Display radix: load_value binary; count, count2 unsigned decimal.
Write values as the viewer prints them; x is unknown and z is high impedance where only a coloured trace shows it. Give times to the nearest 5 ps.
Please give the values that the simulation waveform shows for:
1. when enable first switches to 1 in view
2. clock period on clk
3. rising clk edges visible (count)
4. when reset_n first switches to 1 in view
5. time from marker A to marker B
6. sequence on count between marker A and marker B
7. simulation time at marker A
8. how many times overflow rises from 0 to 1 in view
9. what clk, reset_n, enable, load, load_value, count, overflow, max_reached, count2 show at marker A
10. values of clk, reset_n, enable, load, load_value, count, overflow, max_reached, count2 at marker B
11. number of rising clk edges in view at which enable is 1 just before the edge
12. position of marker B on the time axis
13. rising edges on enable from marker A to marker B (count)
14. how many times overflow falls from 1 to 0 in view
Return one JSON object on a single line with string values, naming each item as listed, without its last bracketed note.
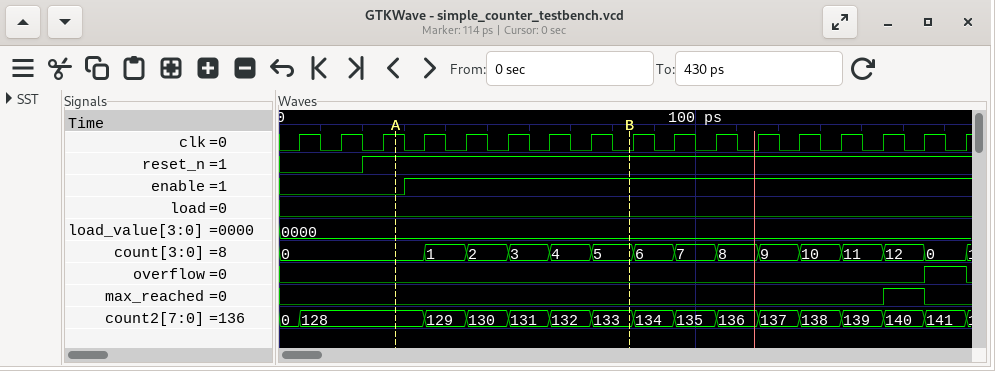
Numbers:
{"when enable first switches to 1 in view": "30 ps", "clock period on clk": "10 ps", "rising clk edges visible": "17", "when reset_n first switches to 1 in view": "20 ps", "time from marker A to marker B": "55 ps", "sequence on count between marker A and marker B": "0, 1, 2, 3, 4, 5", "simulation time at marker A": "30 ps", "how many times overflow rises from 0 to 1 in view": "1", "what clk, reset_n, enable, load, load_value, count, overflow, max_reached, count2 show at marker A": "clk=1, reset_n=1, enable=0, load=0, load_value=0000, count=0, overflow=0, max_reached=0, count2=128", "values of clk, reset_n, enable, load, load_value, count, overflow, max_reached, count2 at marker B": "clk=0, reset_n=1, enable=1, load=0, load_value=0000, count=5, overflow=0, max_reached=0, count2=133", "number of rising clk edges in view at which enable is 1 just before the edge": "14", "position of marker B on the time axis": "85 ps", "rising edges on enable from marker A to marker B": "1", "how many times overflow falls from 1 to 0 in view": "1"}
